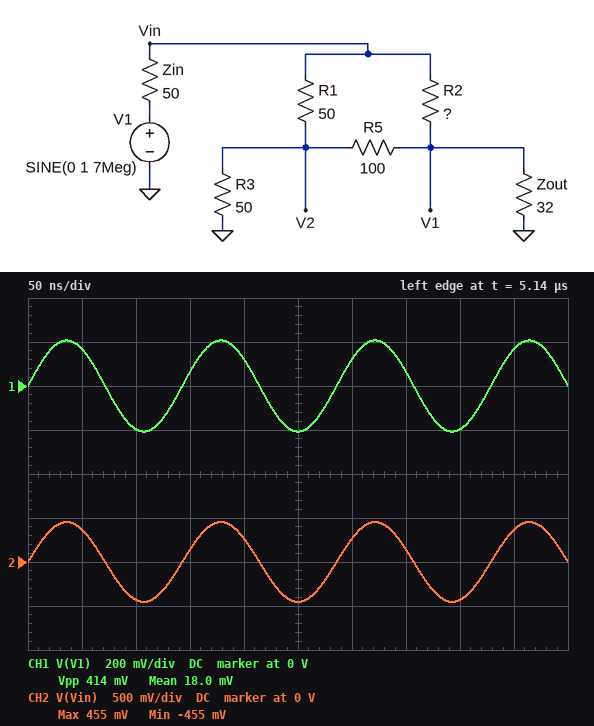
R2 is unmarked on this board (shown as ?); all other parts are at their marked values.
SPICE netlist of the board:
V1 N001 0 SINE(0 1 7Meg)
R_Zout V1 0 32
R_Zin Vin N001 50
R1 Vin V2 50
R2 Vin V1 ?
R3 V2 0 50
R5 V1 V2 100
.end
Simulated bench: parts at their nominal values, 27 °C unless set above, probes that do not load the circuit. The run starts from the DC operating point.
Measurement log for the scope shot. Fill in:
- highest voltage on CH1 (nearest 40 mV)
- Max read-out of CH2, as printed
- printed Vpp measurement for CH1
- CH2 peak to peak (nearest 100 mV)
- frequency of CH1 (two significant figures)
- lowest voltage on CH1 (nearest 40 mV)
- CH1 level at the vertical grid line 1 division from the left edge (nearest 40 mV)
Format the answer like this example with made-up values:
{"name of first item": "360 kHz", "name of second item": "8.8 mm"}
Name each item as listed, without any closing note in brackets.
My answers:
{"highest voltage on CH1": "200 mV", "Max read-out of CH2, as printed": "455 mV", "printed Vpp measurement for CH1": "414 mV", "CH2 peak to peak": "900 mV", "frequency of CH1": "7.0 MHz", "lowest voltage on CH1": "-200 mV", "CH1 level at the vertical grid line 1 division from the left edge": "160 mV"}
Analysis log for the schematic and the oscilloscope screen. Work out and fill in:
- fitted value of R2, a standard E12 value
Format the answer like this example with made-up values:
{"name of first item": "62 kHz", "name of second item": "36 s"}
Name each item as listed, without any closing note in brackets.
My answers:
{"fitted value of R2, a standard E12 value": "39 Ω"}
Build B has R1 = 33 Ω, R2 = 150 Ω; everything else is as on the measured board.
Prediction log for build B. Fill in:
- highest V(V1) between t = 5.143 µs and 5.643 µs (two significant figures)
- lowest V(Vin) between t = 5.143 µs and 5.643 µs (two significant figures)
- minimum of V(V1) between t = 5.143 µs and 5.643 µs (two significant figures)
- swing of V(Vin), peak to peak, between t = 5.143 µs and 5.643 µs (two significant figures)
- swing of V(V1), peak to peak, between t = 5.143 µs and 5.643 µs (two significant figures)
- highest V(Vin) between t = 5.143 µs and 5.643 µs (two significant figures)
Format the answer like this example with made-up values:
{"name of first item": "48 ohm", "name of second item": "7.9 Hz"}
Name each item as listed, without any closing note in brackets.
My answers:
{"highest V(V1) between t = 5.143 µs and 5.643 µs": "130 mV", "lowest V(Vin) between t = 5.143 µs and 5.643 µs": "-520 mV", "minimum of V(V1) between t = 5.143 µs and 5.643 µs": "-130 mV", "swing of V(Vin), peak to peak, between t = 5.143 µs and 5.643 µs": "1.0 V", "swing of V(V1), peak to peak, between t = 5.143 µs and 5.643 µs": "260 mV", "highest V(Vin) between t = 5.143 µs and 5.643 µs": "520 mV"}
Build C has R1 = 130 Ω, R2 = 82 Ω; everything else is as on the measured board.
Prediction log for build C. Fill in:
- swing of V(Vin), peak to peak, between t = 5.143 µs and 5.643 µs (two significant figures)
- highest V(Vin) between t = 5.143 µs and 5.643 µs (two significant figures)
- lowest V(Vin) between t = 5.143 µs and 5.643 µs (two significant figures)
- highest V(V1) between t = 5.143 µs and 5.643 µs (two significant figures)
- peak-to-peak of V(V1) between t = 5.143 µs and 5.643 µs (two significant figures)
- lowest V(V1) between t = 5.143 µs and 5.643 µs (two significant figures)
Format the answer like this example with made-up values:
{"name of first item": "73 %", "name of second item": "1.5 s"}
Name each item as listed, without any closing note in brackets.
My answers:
{"swing of V(Vin), peak to peak, between t = 5.143 µs and 5.643 µs": "1.2 V", "highest V(Vin) between t = 5.143 µs and 5.643 µs": "580 mV", "lowest V(Vin) between t = 5.143 µs and 5.643 µs": "-580 mV", "highest V(V1) between t = 5.143 µs and 5.643 µs": "160 mV", "peak-to-peak of V(V1) between t = 5.143 µs and 5.643 µs": "330 mV", "lowest V(V1) between t = 5.143 µs and 5.643 µs": "-160 mV"}
